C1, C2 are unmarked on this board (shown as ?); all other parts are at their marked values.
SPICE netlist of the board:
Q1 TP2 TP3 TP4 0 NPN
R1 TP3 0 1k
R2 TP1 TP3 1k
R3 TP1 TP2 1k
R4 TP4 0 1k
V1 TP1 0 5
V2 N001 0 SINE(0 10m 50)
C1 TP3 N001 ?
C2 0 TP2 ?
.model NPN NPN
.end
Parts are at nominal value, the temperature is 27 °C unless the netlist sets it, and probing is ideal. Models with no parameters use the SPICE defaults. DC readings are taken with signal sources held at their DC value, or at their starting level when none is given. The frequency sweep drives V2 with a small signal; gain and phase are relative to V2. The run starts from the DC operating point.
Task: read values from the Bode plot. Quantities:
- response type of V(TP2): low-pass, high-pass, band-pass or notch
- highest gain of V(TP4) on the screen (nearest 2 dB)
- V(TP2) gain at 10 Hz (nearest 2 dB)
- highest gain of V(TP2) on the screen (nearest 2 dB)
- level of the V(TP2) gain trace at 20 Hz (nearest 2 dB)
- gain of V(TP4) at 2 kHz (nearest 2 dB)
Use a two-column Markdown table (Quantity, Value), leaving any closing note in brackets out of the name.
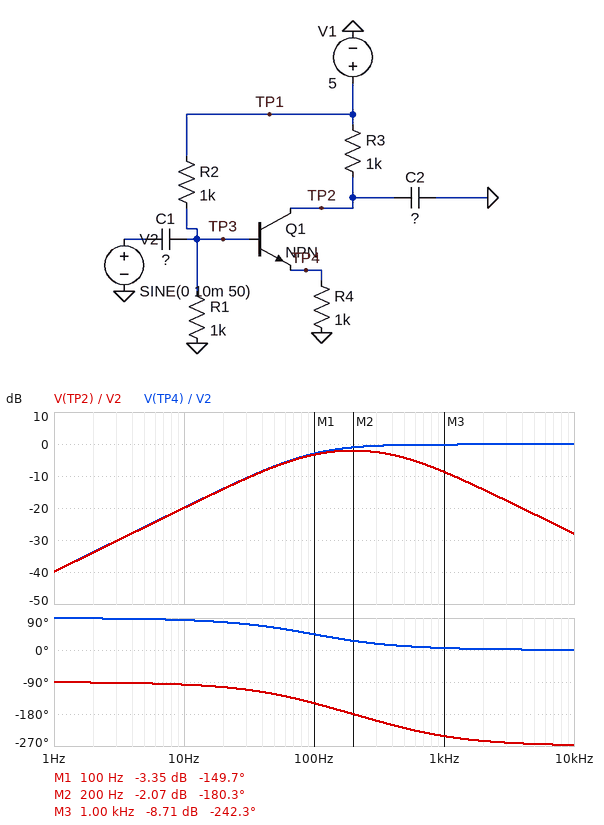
| Quantity | Value |
|---|---|
| response type of V(TP2): low-pass, high-pass, band-pass or notch | band-pass |
| highest gain of V(TP4) on the screen | 0 dB |
| V(TP2) gain at 10 Hz | -20 dB |
| highest gain of V(TP2) on the screen | -2 dB |
| level of the V(TP2) gain trace at 20 Hz | -14 dB |
| gain of V(TP4) at 2 kHz | 0 dB |
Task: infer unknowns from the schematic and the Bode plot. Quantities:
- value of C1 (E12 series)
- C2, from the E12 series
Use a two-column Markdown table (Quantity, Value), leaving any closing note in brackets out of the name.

| Quantity | Value |
|---|---|
| value of C1 | 3.3 µF |
| C2, from the E12 series | 390 nF |
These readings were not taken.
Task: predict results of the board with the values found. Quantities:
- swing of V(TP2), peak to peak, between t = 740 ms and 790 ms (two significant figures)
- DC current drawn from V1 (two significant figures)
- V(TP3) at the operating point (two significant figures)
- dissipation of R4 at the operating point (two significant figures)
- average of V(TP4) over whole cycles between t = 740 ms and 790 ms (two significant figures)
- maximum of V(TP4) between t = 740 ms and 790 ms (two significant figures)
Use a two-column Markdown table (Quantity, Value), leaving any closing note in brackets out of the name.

| Quantity | Value |
|---|---|
| swing of V(TP2), peak to peak, between t = 740 ms and 790 ms | 8.9 mV |
| DC current drawn from V1 | 4.2 mA |
| V(TP3) at the operating point | 2.5 V |
| dissipation of R4 at the operating point | 2.9 mW |
| average of V(TP4) over whole cycles between t = 740 ms and 790 ms | 1.7 V |
| maximum of V(TP4) between t = 740 ms and 790 ms | 1.7 V |
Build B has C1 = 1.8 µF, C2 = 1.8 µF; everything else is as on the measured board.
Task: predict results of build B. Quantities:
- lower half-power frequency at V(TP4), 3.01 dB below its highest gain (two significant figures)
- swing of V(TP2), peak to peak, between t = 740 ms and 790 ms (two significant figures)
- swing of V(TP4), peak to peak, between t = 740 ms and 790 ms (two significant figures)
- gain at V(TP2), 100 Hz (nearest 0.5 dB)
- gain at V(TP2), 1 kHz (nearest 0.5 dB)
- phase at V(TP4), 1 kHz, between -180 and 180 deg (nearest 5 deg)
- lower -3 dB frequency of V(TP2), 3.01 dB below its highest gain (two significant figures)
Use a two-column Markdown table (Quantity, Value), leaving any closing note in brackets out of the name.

| Quantity | Value |
|---|---|
| lower half-power frequency at V(TP4), 3.01 dB below its highest gain | 180 Hz |
| swing of V(TP2), peak to peak, between t = 740 ms and 790 ms | 4.6 mV |
| swing of V(TP4), peak to peak, between t = 740 ms and 790 ms | 5.3 mV |
| gain at V(TP2), 100 Hz | -10.0 dB |
| gain at V(TP2), 1 kHz | -21.5 dB |
| phase at V(TP4), 1 kHz, between -180 and 180 deg | 10 deg |
| lower -3 dB frequency of V(TP2), 3.01 dB below its highest gain | 50 Hz |
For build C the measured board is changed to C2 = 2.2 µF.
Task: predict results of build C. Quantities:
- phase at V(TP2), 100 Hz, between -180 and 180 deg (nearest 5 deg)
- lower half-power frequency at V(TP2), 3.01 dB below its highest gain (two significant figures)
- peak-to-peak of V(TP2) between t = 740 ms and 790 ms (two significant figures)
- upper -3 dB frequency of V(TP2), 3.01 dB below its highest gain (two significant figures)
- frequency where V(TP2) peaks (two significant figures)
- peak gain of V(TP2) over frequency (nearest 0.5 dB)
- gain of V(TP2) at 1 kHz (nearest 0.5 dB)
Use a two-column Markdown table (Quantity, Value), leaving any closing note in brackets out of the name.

| Quantity | Value |
|---|---|
| phase at V(TP2), 100 Hz, between -180 and 180 deg | 170 deg |
| lower half-power frequency at V(TP2), 3.01 dB below its highest gain | 34 Hz |
| peak-to-peak of V(TP2) between t = 740 ms and 790 ms | 7.4 mV |
| upper -3 dB frequency of V(TP2), 3.01 dB below its highest gain | 200 Hz |
| frequency where V(TP2) peaks | 84 Hz |
| peak gain of V(TP2) over frequency | -7.5 dB |
| gain of V(TP2) at 1 kHz | -23.0 dB |
